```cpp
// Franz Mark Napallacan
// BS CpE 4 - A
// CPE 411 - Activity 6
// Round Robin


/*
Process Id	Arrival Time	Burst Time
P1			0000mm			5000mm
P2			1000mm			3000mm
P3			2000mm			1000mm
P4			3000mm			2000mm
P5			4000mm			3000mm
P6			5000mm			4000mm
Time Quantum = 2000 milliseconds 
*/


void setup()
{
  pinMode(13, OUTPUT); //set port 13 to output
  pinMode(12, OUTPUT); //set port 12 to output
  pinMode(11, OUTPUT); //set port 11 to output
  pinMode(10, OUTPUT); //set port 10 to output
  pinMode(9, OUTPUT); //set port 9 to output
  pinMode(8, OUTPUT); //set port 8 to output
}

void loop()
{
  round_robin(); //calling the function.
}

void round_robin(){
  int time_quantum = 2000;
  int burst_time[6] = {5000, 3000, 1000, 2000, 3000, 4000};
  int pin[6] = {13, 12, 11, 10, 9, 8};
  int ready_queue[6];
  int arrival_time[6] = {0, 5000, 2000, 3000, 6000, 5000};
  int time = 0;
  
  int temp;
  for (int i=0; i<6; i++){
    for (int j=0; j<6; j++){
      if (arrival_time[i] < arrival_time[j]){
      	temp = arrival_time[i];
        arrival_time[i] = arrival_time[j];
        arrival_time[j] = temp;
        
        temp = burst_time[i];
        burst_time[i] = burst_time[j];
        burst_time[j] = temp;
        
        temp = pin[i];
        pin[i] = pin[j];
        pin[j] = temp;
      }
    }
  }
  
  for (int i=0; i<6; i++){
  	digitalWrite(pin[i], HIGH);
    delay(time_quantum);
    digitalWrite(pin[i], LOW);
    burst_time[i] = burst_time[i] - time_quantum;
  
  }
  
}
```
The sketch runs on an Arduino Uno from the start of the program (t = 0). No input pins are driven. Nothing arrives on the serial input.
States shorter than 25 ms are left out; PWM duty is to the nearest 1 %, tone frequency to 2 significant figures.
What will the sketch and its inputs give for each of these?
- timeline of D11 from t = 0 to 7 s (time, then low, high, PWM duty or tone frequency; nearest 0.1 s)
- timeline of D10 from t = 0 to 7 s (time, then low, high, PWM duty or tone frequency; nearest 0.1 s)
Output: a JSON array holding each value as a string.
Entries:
["0 s low; 2 s high; 4 s low", "0 s low; 4 s high; 6 s low"]
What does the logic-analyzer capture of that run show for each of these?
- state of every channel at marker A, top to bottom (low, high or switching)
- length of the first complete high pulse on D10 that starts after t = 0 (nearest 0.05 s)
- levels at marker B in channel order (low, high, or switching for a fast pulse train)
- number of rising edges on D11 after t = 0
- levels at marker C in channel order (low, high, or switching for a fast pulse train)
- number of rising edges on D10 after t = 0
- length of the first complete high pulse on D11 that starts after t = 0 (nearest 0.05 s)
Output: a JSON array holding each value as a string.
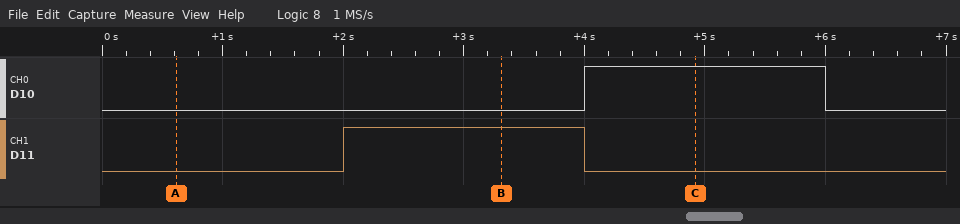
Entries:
["D10 low, D11 low", "2.00 s", "D10 low, D11 high", "1", "D10 high, D11 low", "1", "2.00 s"]
